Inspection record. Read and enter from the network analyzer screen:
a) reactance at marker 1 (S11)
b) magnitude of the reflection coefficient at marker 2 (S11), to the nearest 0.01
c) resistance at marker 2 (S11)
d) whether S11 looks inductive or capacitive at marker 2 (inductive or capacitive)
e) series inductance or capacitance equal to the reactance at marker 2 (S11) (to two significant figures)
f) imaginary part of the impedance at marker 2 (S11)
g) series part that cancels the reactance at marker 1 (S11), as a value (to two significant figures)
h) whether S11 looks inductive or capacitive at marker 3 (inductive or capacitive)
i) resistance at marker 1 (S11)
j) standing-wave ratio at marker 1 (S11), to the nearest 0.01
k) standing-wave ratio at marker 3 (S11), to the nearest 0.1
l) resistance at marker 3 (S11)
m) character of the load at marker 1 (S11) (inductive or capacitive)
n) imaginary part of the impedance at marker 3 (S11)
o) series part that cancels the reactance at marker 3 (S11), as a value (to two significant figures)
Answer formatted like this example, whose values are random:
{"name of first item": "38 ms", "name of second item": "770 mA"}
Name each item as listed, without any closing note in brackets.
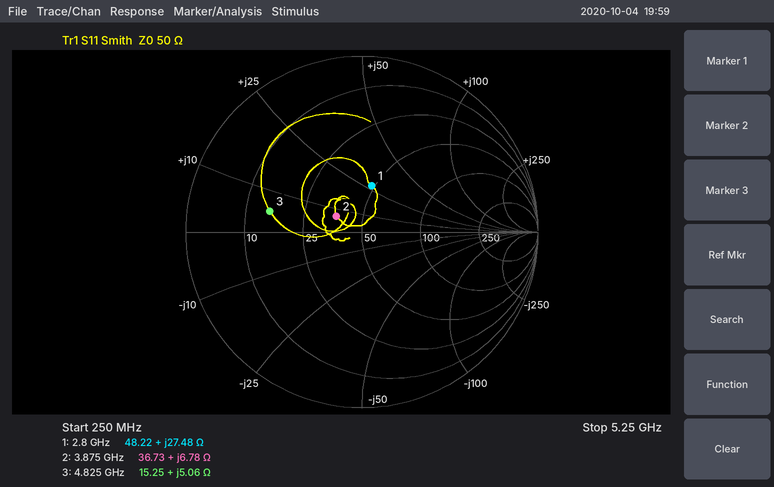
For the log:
{"reactance at marker 1": "+27.48 Ω", "magnitude of the reflection coefficient at marker 2 (S11), to the nearest 0.01": "0.17", "resistance at marker 2": "36.73 Ω", "whether S11 looks inductive or capacitive at marker 2": "inductive", "series inductance or capacitance equal to the reactance at marker 2 (S11)": "280 pH", "imaginary part of the impedance at marker 2": "+6.78 Ω", "series part that cancels the reactance at marker 1 (S11), as a value": "2.1 pF", "whether S11 looks inductive or capacitive at marker 3": "inductive", "resistance at marker 1": "48.22 Ω", "standing-wave ratio at marker 1 (S11), to the nearest 0.01": "1.74", "standing-wave ratio at marker 3 (S11), to the nearest 0.1": "3.3", "resistance at marker 3": "15.25 Ω", "character of the load at marker 1 (S11)": "inductive", "imaginary part of the impedance at marker 3": "+5.06 Ω", "series part that cancels the reactance at marker 3 (S11), as a value": "6.5 pF"}
